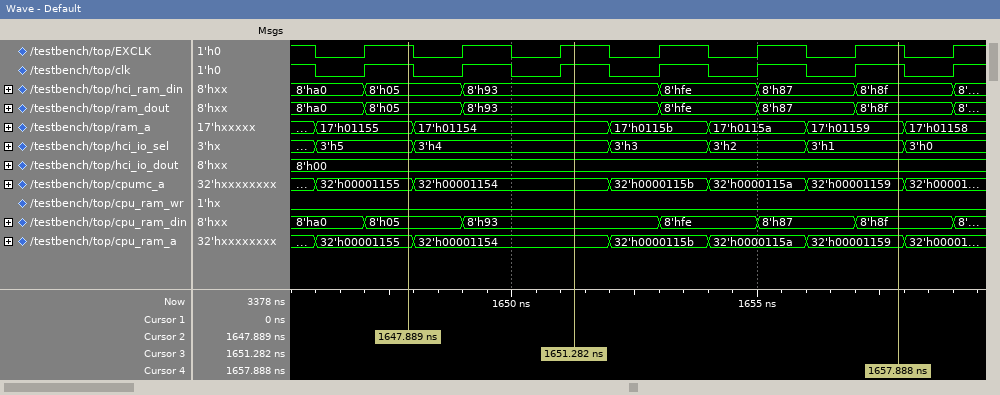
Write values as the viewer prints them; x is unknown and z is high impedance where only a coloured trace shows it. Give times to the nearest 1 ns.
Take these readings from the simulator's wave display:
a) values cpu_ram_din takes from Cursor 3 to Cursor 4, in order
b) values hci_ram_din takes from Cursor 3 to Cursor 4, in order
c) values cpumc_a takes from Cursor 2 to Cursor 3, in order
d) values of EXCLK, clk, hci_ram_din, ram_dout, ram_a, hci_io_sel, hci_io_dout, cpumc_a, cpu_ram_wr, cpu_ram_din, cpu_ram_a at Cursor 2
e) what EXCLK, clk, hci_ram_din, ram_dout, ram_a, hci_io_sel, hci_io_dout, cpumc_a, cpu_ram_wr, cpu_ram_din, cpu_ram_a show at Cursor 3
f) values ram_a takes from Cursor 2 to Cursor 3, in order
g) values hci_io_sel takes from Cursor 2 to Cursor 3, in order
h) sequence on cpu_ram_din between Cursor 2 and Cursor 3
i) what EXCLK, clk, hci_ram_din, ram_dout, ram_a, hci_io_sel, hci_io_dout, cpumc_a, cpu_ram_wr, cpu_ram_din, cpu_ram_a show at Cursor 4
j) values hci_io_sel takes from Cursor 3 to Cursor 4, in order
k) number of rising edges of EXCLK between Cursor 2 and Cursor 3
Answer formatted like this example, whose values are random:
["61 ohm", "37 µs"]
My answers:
["8'h93, 8'hfe, 8'h87, 8'h8f", "8'h93, 8'hfe, 8'h87, 8'h8f", "32'h00001155, 32'h00001154", "EXCLK=1, clk=1, hci_ram_din=8'h05, ram_dout=8'h05, ram_a=17'h01155, hci_io_sel=3'h5, hci_io_dout=8'h00, cpumc_a=32'h00001155, cpu_ram_wr=0, cpu_ram_din=8'h05, cpu_ram_a=32'h00001155", "EXCLK=1, clk=1, hci_ram_din=8'h93, ram_dout=8'h93, ram_a=17'h01154, hci_io_sel=3'h4, hci_io_dout=8'h00, cpumc_a=32'h00001154, cpu_ram_wr=0, cpu_ram_din=8'h93, cpu_ram_a=32'h00001154", "17'h01155, 17'h01154", "3'h5, 3'h4", "8'h05, 8'h93", "EXCLK=1, clk=1, hci_ram_din=8'h8f, ram_dout=8'h8f, ram_a=17'h01159, hci_io_sel=3'h1, hci_io_dout=8'h00, cpumc_a=32'h00001159, cpu_ram_wr=0, cpu_ram_din=8'h8f, cpu_ram_a=32'h00001159", "3'h4, 3'h3, 3'h2, 3'h1", "2"]
